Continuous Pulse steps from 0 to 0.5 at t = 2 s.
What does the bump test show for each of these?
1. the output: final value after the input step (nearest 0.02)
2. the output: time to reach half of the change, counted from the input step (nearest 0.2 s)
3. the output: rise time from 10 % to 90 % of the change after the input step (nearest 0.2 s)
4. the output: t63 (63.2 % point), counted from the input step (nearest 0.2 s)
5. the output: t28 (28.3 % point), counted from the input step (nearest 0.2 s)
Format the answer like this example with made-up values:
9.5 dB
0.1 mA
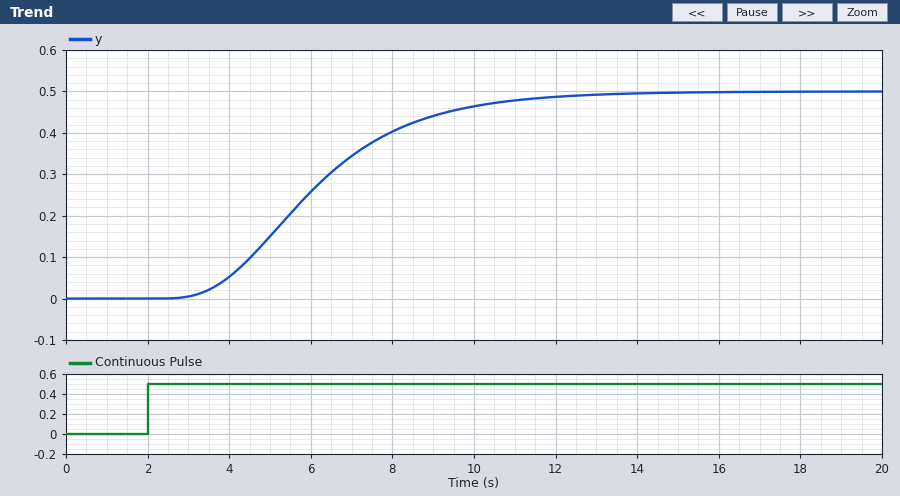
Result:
0.50
4.0 s
5.4 s
4.6 s
3.0 s
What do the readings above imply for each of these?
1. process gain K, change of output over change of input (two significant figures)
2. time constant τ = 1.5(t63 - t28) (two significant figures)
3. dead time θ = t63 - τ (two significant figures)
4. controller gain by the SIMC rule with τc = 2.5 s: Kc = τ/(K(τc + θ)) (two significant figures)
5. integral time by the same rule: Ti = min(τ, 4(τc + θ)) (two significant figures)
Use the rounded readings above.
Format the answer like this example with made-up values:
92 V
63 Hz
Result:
1.0
2.4 s
2.2 s
0.51
2.4 s
